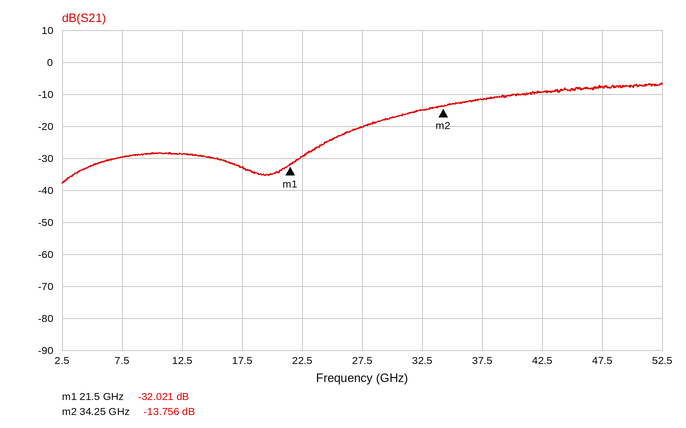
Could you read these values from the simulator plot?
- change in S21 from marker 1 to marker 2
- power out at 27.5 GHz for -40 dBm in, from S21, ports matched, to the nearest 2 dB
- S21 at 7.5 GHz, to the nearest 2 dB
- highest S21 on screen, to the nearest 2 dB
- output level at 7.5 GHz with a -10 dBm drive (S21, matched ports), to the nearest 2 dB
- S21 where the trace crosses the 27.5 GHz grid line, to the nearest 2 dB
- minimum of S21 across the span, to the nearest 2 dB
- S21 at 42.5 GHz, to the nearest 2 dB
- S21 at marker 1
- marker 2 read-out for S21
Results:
18.265 dB
-60 dBm
-30 dB
-6 dB
-40 dBm
-20 dB
-38 dB
-10 dB
-32.021 dB
-13.756 dB
